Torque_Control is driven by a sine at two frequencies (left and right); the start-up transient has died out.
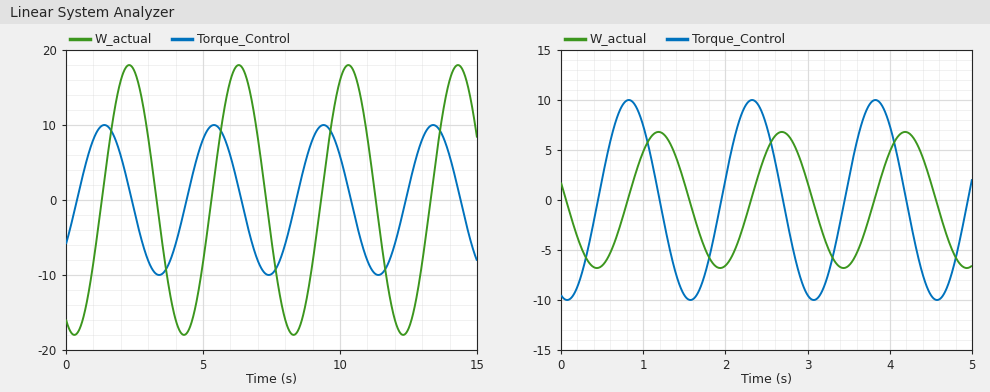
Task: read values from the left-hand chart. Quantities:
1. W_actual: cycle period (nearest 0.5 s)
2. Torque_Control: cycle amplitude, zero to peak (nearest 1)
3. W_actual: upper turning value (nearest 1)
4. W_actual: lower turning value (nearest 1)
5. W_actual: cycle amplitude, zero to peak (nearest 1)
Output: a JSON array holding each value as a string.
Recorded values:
["4.0 s", "10", "18", "-18", "18"]
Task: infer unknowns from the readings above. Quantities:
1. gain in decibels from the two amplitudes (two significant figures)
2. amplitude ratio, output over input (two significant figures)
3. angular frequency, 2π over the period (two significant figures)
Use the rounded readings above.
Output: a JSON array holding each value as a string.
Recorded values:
["5.1 dB", "1.8", "1.6 rad/s"]
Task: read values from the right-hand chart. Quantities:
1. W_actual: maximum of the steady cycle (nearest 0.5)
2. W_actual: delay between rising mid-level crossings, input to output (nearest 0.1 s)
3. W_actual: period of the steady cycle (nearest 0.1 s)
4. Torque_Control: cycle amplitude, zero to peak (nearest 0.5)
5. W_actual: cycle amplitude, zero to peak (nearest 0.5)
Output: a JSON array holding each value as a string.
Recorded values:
["7.0", "0.4 s", "1.5 s", "10.0", "7.0"]
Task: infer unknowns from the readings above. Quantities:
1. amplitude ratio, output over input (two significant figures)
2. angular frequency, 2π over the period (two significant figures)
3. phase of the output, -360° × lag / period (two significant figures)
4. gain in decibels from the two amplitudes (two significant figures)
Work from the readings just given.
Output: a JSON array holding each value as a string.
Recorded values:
["0.70", "4.2 rad/s", "-96°", "-3.1 dB"]
